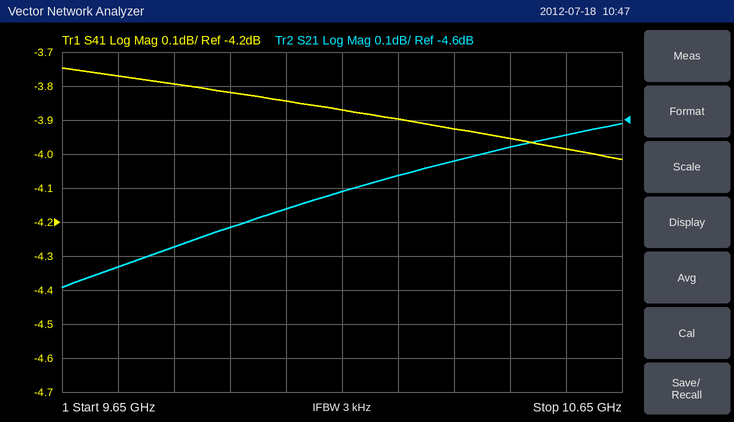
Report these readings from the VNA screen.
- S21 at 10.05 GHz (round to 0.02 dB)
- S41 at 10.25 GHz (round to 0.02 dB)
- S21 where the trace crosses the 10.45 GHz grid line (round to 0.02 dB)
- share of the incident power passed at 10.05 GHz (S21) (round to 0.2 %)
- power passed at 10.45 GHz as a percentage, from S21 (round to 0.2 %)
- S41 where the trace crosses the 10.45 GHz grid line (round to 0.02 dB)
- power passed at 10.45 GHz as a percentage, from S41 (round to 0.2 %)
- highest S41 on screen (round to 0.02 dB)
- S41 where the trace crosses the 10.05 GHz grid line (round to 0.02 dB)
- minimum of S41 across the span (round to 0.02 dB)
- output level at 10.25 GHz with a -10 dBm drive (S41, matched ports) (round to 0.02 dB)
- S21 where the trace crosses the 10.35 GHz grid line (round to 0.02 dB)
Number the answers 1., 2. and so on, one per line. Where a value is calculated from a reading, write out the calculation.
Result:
1. -4.86 dB
2. -3.90 dB
3. -4.68 dB
4. 10^(-4.86/10) ≈ 32.7 %, so 32.6 % to the nearest 0.2 %
5. 10^(-4.68/10) ≈ 34.0 %
6. -3.96 dB
7. 10^(-3.96/10) ≈ 40.2 %
8. -3.74 dB
9. -3.84 dB
10. -4.02 dB
11. -10 dBm + (-3.90 dB) = -13.90 dBm
12. -4.72 dB
